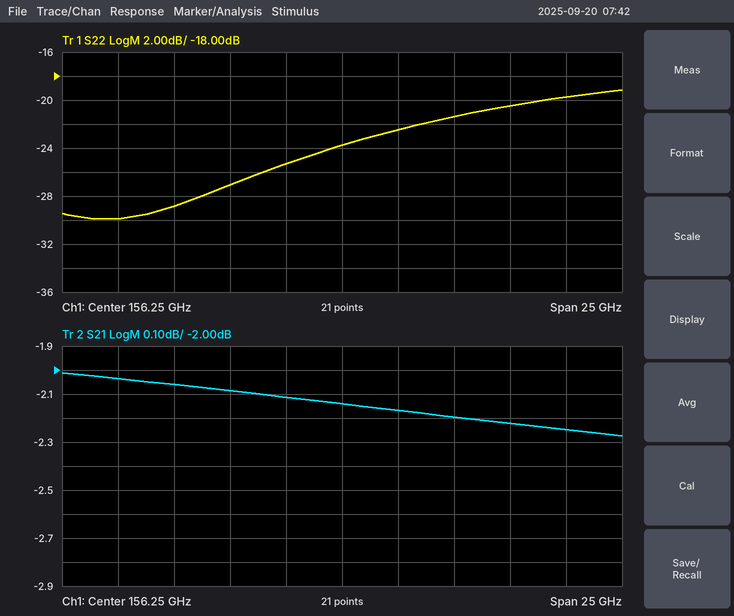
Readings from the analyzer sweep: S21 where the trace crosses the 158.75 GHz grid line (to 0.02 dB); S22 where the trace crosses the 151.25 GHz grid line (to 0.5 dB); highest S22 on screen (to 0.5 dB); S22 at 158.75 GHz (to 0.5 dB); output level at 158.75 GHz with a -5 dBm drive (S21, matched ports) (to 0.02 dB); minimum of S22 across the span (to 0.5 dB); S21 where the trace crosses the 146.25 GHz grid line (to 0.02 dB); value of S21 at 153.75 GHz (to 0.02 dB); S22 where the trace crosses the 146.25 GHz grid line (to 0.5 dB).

-2.16 dB
-27.0 dB
-19.0 dB
-22.5 dB
-7.16 dBm
-30.0 dB
-2.04 dB
-2.12 dB
-30.0 dB
